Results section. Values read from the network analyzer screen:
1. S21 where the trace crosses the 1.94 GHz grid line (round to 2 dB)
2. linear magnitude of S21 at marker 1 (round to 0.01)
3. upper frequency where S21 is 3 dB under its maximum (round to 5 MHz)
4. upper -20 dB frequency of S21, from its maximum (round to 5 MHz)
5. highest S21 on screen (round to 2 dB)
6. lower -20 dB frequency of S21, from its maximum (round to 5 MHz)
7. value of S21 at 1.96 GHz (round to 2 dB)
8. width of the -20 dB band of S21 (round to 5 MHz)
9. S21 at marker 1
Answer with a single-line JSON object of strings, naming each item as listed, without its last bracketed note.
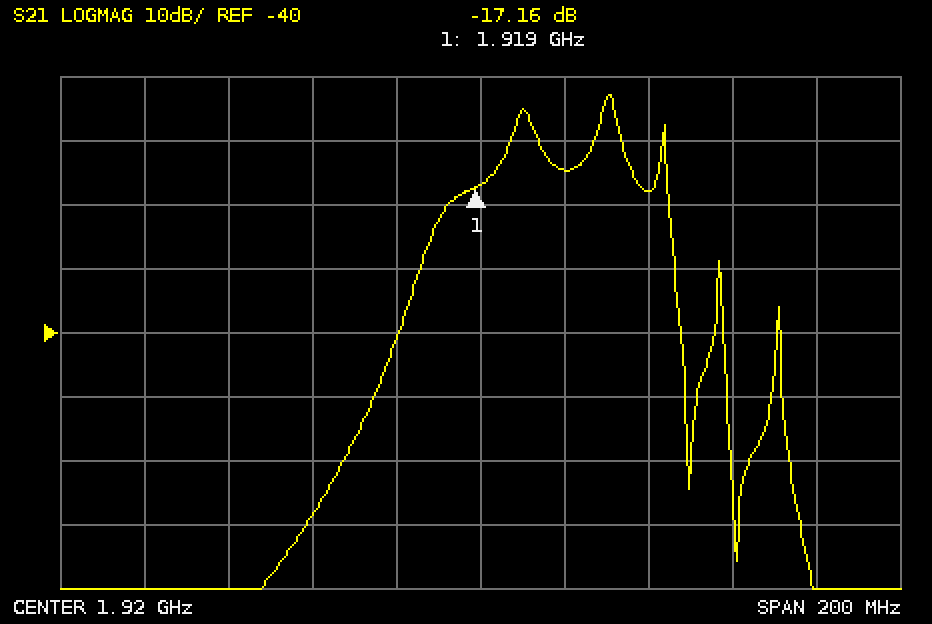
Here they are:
{"S21 where the trace crosses the 1.94 GHz grid line": "-14 dB", "linear magnitude of S21 at marker 1": "0.14", "upper frequency where S21 is 3 dB under its maximum": "1.950 GHz", "upper -20 dB frequency of S21, from its maximum": "1.965 GHz", "highest S21 on screen": "-2 dB", "lower -20 dB frequency of S21, from its maximum": "1.910 GHz", "value of S21 at 1.96 GHz": "-18 dB", "width of the -20 dB band of S21": "55 MHz", "S21 at marker 1": "-17.16 dB"}
